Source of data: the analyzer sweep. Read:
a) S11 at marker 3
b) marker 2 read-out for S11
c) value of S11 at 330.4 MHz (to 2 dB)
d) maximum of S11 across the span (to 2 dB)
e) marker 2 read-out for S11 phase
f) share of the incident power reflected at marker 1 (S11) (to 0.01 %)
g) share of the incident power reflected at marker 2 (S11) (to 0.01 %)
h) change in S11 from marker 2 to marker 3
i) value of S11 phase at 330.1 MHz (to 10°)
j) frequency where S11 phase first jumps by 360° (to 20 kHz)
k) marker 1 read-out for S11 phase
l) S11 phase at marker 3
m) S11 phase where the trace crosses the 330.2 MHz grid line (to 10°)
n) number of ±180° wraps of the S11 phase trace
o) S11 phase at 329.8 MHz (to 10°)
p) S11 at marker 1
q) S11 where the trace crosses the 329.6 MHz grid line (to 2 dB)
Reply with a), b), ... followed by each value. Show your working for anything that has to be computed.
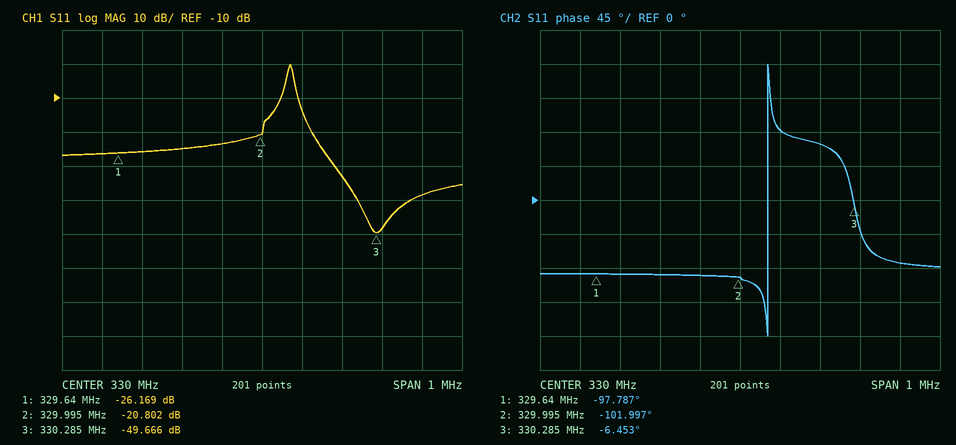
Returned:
a) -49.666 dB
b) -20.802 dB
c) -38 dB
d) 0 dB
e) -101.997°
f) 10^(-26.169/10) ≈ 0.24 %
g) 10^(-20.802/10) ≈ 0.83 %
h) -49.666 − (-20.802) = -28.864 dB
i) 90°
j) 330.06 MHz
k) -97.787°
l) -6.453°
m) 70°
n) 1
o) -100°
p) -26.169 dB
q) -26 dB
